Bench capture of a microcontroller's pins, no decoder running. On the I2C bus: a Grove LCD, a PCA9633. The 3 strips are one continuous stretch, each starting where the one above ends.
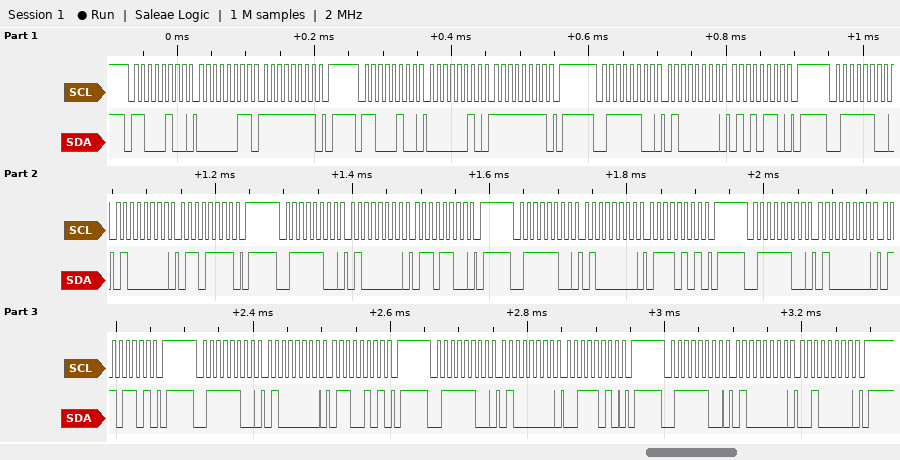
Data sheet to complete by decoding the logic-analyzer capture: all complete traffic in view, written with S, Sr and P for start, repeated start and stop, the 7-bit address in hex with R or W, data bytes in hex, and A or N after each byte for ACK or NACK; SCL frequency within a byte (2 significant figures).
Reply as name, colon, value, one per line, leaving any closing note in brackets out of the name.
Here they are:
all complete traffic in view, written with S, Sr and P for start, repeated start and stop, the 7-bit address in hex with R or W, data bytes in hex, and A or N after each byte for ACK or NACK: S 62W A 03 A FF A P S 62W A 02 A FF A P S 3EW A 40 A 56 A P S 3EW A 40 A 6F A P S 3EW A 40 A 6C A P S 3EW A 40 A 75 A P S 3EW A 40 A 6D A P S 3EW A 40 A 65 A P S 3EW A 40 A 3A A P S 3EW A 40 A 20 A P
SCL frequency within a byte: 100 kHz
